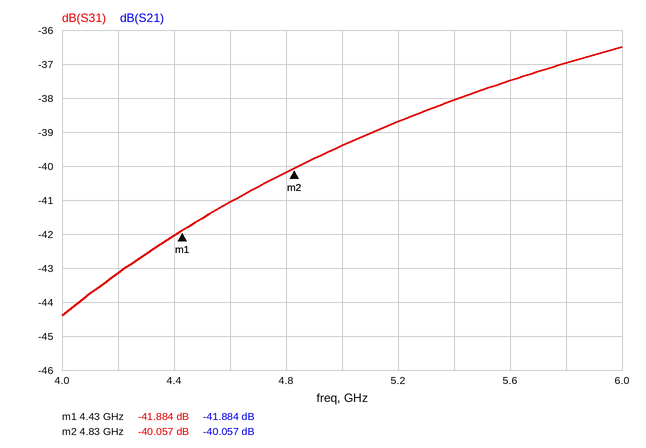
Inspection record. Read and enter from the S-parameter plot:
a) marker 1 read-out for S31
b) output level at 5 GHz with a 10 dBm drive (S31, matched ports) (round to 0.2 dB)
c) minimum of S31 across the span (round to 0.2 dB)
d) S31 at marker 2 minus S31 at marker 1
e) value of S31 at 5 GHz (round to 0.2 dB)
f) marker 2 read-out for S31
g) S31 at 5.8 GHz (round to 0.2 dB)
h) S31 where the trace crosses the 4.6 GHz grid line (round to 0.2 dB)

-41.884 dB
-29.4 dBm
-44.4 dB
1.827 dB
-39.4 dB
-40.057 dB
-37.0 dB
-41.0 dB
